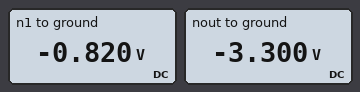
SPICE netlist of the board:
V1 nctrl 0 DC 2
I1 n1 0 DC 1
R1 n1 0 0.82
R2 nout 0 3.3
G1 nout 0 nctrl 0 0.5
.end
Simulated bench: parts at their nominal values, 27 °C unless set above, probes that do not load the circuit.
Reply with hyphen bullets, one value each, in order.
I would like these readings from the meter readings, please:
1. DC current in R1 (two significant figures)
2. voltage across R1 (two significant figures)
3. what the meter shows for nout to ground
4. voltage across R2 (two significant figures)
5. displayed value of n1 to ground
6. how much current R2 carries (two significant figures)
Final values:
- 1.0 A
- 820 mV
- -3.300 V
- 3.3 V
- -0.820 V
- 1.0 A
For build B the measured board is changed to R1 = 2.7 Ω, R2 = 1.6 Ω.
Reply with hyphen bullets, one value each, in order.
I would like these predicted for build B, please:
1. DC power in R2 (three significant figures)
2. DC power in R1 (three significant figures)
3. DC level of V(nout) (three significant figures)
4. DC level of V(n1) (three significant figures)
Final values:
- 1.60 W
- 2.70 W
- -1.60 V
- -2.70 V
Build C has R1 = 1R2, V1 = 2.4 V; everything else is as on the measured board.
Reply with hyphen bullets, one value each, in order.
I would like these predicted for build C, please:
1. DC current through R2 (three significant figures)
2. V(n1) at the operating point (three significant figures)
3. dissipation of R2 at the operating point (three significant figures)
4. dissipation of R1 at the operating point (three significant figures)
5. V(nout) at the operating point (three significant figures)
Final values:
- 1.20 A
- -1.20 V
- 4.75 W
- 1.20 W
- -3.96 V
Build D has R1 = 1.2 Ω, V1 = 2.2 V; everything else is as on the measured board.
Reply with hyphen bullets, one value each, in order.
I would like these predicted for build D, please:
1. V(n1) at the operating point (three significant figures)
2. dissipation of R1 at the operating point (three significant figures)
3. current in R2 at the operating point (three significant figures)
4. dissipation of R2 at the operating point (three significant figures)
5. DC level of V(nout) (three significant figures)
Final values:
- -1.20 V
- 1.20 W
- 1.10 A
- 3.99 W
- -3.63 V
